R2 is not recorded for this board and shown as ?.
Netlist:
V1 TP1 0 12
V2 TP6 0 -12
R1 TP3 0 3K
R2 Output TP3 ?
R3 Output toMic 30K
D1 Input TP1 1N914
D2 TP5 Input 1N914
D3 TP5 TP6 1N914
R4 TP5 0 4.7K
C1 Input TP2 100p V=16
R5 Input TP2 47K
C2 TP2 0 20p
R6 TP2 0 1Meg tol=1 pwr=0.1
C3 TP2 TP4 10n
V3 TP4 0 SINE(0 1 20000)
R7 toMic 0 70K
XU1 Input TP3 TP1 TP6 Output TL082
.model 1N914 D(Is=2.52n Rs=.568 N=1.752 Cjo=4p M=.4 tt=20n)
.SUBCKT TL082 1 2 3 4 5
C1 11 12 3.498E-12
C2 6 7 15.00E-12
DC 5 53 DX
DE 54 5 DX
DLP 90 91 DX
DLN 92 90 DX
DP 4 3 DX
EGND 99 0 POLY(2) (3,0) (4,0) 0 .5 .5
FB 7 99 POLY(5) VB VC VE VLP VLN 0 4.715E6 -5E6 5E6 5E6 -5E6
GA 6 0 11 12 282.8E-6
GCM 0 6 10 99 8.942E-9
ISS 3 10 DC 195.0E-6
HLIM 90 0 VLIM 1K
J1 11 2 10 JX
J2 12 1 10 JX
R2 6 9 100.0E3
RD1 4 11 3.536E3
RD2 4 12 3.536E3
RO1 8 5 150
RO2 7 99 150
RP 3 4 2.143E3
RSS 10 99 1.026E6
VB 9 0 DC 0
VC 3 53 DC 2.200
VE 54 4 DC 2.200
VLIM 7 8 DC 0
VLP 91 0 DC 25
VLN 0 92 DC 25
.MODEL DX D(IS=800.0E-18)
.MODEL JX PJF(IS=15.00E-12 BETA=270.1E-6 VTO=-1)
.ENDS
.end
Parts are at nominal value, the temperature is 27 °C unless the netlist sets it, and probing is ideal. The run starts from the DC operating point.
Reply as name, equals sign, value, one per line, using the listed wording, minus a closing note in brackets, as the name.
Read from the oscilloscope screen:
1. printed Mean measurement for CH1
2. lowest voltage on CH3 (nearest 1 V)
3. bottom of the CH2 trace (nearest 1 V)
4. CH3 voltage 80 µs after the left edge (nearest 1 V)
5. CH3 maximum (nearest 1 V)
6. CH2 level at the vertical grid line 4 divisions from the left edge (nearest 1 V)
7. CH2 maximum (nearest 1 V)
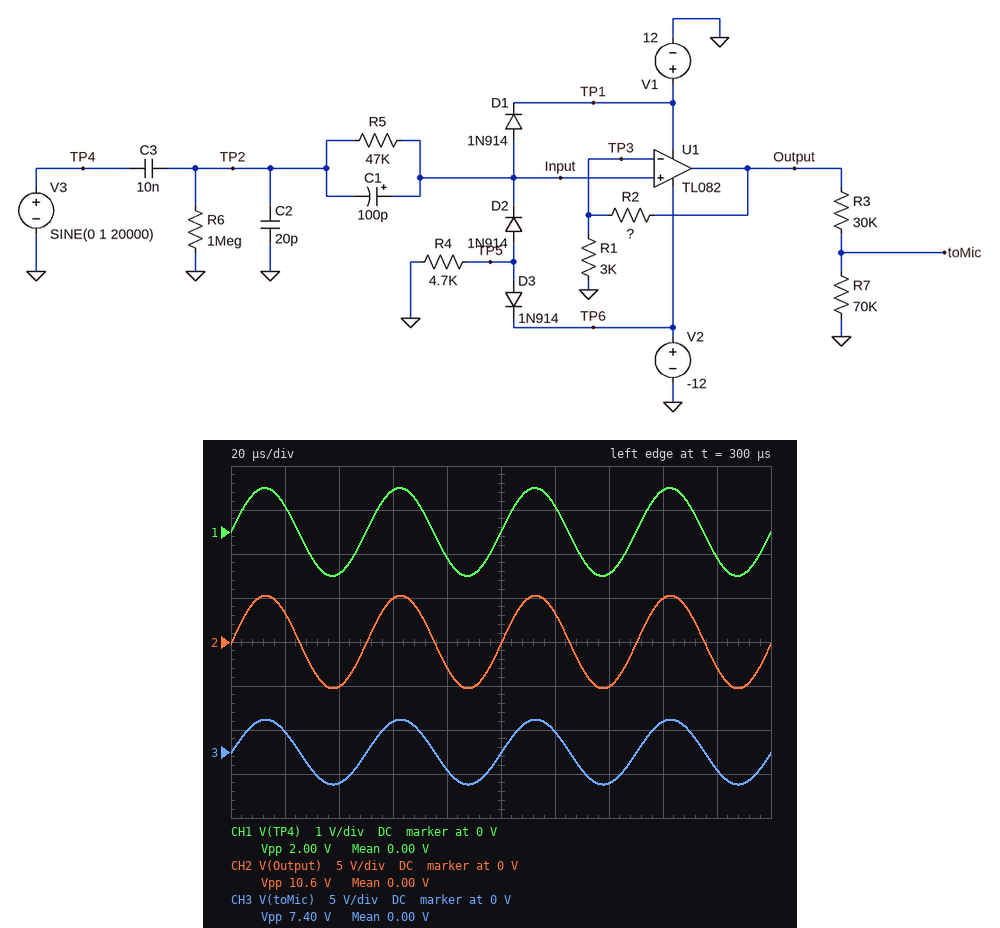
printed Mean measurement for CH1 = 0.00 V
lowest voltage on CH3 = -4 V
bottom of the CH2 trace = -5 V
CH3 voltage 80 µs after the left edge = -2 V
CH3 maximum = 4 V
CH2 level at the vertical grid line 4 divisions from the left edge = -3 V
CH2 maximum = 5 V
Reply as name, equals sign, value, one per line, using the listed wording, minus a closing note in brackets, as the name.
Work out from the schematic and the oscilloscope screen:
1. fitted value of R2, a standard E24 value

fitted value of R2, a standard E24 value = 13 kΩ
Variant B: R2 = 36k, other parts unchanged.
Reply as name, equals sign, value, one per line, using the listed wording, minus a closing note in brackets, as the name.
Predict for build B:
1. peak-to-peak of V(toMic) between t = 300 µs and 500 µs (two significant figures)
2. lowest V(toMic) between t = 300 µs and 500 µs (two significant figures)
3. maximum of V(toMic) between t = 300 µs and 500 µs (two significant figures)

peak-to-peak of V(toMic) between t = 300 µs and 500 µs = 15 V
lowest V(toMic) between t = 300 µs and 500 µs = -7.3 V
maximum of V(toMic) between t = 300 µs and 500 µs = 7.3 V
